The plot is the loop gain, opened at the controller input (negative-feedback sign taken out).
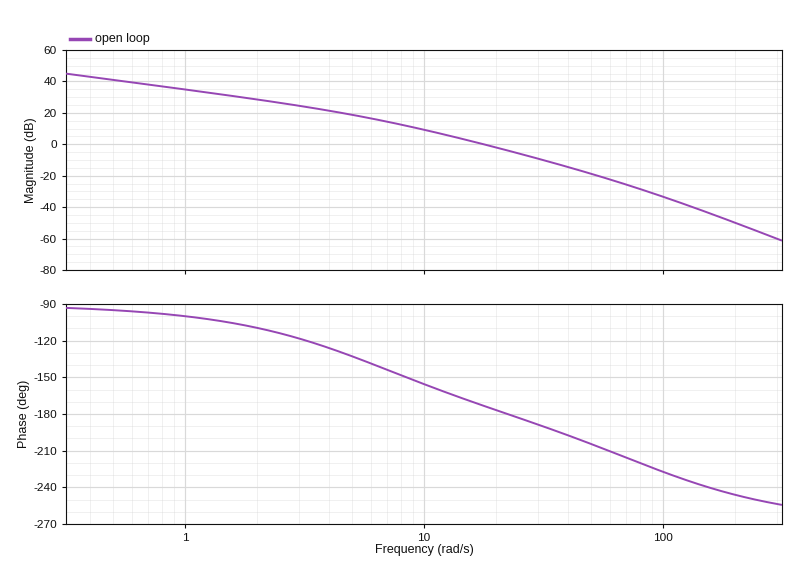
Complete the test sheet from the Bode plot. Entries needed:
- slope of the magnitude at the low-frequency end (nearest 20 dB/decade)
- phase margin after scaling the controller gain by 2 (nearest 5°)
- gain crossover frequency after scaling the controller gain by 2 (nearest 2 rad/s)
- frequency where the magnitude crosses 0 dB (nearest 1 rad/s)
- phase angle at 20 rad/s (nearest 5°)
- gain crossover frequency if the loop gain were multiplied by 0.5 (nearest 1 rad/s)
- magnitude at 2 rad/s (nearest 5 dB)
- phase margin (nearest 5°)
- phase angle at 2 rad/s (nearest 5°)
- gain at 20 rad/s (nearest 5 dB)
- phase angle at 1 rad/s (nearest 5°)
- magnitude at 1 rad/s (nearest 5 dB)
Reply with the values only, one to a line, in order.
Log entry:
-20 dB/decade
-5°
26 rad/s
18 rad/s
-175°
12 rad/s
30 dB
5°
-110°
0 dB
-100°
35 dB
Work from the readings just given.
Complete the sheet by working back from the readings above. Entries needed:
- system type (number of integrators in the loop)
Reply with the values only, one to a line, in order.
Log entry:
1
